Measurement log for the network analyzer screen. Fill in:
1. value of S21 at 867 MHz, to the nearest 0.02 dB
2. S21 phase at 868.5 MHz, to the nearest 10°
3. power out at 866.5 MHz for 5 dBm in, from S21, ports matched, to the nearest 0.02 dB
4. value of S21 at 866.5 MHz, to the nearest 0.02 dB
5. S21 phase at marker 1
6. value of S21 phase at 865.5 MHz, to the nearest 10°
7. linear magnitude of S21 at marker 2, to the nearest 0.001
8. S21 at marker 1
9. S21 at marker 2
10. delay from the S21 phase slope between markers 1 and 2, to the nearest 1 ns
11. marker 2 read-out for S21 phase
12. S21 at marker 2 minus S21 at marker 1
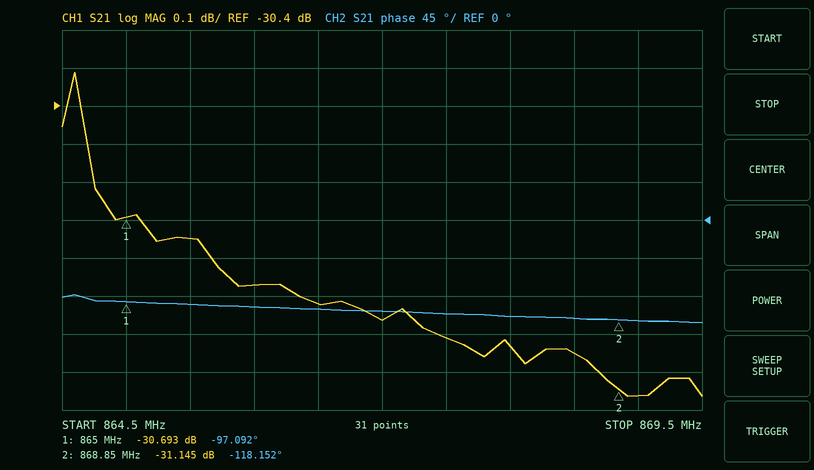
-30.96 dB
-120°
-25.92 dBm
-30.92 dB
-97.092°
-100°
0.028
-30.693 dB
-31.145 dB
15 ns
-118.152°
-0.452 dB
